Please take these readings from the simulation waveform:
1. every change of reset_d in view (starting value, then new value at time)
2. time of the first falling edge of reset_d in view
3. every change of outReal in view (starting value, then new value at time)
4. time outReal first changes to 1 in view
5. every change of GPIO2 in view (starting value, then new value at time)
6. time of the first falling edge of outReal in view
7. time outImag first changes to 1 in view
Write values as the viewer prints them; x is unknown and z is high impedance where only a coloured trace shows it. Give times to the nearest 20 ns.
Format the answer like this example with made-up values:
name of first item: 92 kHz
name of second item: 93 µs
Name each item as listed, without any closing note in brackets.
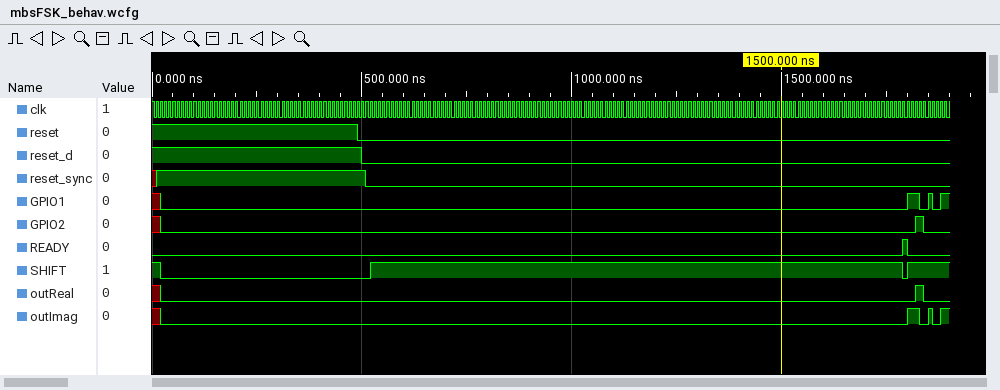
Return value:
every change of reset_d in view: 1, 0 at 500 ns
time of the first falling edge of reset_d in view: 500 ns
every change of outReal in view: x, 0 at 20 ns, 1 at 1820 ns, 0 at 1840 ns
time outReal first changes to 1 in view: 1820 ns
every change of GPIO2 in view: x, 0 at 20 ns, 1 at 1820 ns, 0 at 1840 ns
time of the first falling edge of outReal in view: 1840 ns
time outImag first changes to 1 in view: 1800 ns
